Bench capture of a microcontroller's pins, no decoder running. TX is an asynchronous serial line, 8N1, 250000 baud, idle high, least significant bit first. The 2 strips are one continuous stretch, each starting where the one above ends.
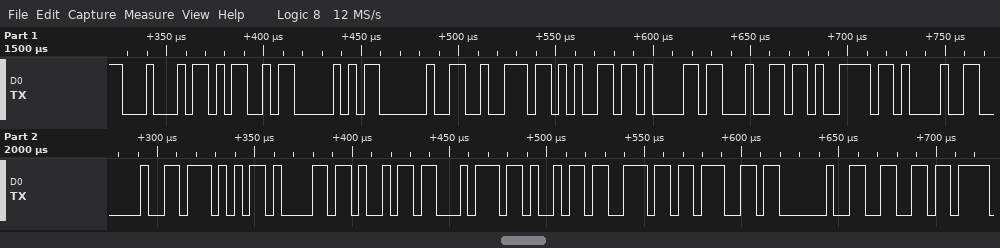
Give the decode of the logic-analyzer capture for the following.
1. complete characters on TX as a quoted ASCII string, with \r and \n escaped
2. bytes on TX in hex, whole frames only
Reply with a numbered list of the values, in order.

1. "DMP ready! Waiting f"
2. 44 4D 50 20 72 65 61 64 79 21 20 57 61 69 74 69 6E 67 20 66
